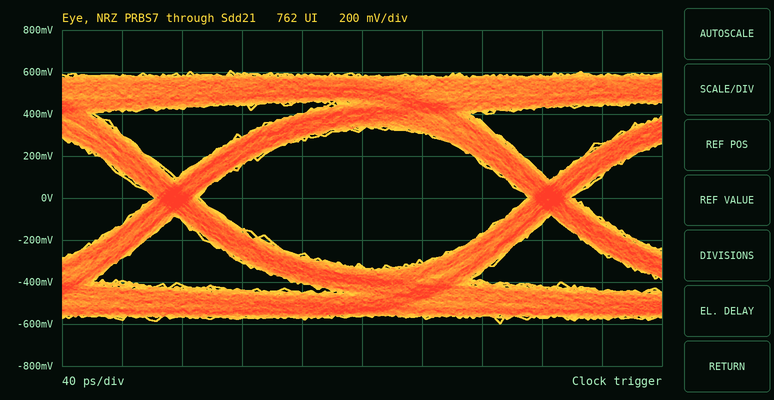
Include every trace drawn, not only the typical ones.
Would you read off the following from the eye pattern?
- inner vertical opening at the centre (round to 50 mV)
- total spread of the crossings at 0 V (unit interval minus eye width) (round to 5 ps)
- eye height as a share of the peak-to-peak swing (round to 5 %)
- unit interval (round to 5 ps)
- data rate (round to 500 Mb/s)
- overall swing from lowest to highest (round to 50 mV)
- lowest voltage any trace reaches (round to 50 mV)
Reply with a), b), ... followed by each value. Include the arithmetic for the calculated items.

a) 650 mV
b) 30 ps
c) 650 mV / 1.20 V ≈ 54.2 %, so 55 % to the nearest 5 %
d) 250 ps
e) 4.0 Gb/s
f) 1.20 V
g) -600 mV
